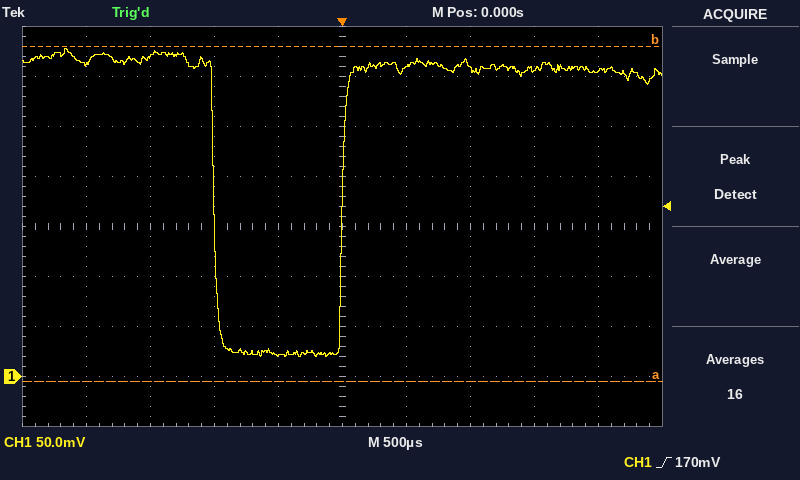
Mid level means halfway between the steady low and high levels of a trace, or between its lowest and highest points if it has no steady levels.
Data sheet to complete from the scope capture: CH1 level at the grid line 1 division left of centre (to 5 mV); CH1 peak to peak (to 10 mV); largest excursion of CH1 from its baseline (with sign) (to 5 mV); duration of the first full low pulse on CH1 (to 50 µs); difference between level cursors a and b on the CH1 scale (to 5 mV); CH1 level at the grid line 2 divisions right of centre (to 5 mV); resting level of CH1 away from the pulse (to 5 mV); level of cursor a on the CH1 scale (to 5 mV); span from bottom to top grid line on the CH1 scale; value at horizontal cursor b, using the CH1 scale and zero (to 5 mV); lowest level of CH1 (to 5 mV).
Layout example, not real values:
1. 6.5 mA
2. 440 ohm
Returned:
1. 20 mV
2. 310 mV
3. -290 mV
4. 1.00 ms
5. 335 mV
6. 310 mV
7. 310 mV
8. -5 mV
9. 400 mV
10. 330 mV
11. 20 mV
